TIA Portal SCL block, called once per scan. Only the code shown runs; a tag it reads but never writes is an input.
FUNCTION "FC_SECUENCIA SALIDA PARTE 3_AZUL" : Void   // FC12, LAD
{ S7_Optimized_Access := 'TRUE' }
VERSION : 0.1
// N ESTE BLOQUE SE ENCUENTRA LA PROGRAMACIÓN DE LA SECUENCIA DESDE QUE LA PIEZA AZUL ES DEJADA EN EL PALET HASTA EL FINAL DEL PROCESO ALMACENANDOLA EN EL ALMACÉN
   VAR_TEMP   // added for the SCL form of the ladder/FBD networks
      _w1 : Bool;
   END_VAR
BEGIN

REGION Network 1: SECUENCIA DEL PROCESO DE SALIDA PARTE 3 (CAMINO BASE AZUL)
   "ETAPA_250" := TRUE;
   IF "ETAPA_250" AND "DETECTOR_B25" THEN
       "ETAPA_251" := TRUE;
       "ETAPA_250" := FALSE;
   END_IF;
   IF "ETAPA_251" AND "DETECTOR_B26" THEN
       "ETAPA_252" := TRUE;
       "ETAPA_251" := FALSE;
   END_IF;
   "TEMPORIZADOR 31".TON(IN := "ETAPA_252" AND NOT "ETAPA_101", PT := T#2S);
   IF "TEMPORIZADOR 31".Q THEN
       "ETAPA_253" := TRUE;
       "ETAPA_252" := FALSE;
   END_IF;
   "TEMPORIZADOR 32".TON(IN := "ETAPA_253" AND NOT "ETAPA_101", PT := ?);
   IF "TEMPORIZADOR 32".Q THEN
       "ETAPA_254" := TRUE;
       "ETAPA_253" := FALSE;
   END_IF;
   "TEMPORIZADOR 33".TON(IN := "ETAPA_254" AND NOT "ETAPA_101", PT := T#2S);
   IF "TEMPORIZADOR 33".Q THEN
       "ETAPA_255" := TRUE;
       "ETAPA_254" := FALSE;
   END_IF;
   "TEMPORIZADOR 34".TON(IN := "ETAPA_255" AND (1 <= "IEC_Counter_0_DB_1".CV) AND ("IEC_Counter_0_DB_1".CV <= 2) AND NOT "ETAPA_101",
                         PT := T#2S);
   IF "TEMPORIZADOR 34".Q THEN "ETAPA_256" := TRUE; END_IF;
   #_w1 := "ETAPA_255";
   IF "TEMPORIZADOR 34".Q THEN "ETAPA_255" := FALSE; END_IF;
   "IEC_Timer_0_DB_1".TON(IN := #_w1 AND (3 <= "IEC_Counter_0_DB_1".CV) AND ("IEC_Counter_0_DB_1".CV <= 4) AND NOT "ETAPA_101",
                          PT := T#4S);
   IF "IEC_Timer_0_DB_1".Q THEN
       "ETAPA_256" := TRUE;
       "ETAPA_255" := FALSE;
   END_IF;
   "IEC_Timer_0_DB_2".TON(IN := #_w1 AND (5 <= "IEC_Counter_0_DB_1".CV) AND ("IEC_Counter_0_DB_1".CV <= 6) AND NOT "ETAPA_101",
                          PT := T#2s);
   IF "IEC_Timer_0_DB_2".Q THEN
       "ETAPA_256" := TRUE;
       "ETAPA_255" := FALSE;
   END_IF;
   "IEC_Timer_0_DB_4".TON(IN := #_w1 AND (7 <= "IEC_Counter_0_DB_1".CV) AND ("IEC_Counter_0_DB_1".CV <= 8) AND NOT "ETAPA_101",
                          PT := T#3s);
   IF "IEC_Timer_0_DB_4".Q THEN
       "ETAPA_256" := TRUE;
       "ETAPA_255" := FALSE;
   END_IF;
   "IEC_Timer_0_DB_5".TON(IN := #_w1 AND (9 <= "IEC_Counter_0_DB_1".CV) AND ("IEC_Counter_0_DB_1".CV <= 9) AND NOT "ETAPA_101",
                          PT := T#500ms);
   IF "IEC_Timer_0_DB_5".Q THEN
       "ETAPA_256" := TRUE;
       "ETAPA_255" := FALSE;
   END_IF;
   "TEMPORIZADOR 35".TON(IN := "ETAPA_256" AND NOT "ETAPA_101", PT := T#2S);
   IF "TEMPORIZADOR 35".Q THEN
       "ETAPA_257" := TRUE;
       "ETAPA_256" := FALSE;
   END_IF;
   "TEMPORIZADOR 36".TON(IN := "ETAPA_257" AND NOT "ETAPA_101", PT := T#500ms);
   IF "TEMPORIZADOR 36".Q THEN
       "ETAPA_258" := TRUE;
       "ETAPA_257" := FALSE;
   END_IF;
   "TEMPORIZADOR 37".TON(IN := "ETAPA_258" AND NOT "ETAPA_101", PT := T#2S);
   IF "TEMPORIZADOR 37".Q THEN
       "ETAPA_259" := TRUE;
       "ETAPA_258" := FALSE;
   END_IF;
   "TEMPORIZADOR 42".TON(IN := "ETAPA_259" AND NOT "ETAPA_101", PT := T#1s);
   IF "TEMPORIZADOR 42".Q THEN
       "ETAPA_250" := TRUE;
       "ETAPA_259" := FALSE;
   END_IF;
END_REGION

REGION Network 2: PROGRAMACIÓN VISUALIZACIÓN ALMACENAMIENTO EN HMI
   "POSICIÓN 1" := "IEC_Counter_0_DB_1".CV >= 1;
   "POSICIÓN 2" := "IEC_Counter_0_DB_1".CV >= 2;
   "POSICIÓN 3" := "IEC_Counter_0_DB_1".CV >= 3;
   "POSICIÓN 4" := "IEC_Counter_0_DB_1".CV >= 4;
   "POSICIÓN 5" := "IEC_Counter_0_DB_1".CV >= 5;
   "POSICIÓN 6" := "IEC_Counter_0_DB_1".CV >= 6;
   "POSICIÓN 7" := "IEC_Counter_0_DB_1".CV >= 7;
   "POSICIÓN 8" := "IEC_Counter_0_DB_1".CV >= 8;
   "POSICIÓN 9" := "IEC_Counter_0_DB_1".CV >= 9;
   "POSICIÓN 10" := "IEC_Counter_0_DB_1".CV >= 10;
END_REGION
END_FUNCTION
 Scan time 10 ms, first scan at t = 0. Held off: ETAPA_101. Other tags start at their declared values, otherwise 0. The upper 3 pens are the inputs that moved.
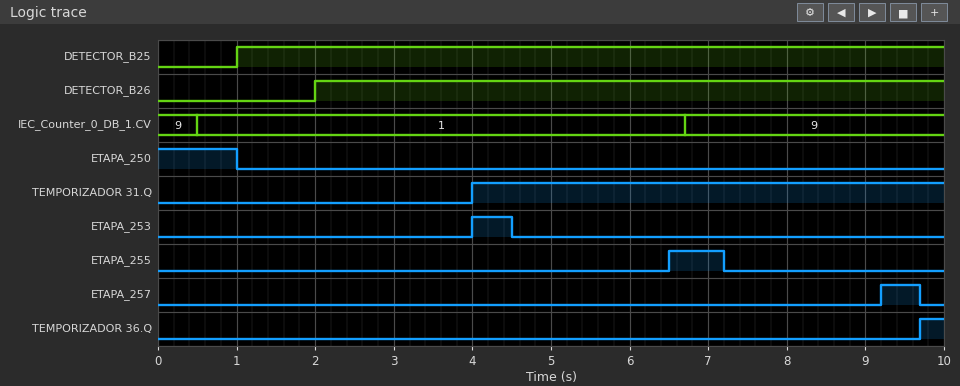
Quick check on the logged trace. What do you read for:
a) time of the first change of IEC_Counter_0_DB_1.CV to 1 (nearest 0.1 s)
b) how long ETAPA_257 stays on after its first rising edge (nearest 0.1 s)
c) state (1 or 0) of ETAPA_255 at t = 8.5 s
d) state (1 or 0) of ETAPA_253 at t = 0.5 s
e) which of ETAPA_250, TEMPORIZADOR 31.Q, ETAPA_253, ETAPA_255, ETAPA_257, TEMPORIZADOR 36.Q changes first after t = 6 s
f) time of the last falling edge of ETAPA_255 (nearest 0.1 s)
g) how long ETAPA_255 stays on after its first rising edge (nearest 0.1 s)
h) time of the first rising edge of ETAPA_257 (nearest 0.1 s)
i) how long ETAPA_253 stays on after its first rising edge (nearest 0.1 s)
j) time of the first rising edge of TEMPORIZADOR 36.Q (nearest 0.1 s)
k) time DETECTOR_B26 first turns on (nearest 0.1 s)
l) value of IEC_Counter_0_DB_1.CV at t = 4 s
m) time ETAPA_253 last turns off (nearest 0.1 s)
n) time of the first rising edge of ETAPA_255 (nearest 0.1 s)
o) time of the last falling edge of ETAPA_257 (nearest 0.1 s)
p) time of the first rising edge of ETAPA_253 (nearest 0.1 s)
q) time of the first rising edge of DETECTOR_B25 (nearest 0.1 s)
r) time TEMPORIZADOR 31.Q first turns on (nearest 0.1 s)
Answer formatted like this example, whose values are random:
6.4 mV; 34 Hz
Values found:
0.5 s; 0.5 s; 0; 0; ETAPA_255; 7.2 s; 0.7 s; 9.2 s; 0.5 s; 9.7 s; 2.0 s; 1; 4.5 s; 6.5 s; 9.7 s; 4.0 s; 1.0 s; 4.0 s
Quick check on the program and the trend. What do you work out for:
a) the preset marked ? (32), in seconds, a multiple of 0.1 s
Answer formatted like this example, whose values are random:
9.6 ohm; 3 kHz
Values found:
0.5 s
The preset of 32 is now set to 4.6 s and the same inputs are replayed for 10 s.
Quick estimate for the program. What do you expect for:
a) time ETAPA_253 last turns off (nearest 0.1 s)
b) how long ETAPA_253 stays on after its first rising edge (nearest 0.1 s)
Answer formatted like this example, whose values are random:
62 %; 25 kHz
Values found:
8.6 s; 4.6 s
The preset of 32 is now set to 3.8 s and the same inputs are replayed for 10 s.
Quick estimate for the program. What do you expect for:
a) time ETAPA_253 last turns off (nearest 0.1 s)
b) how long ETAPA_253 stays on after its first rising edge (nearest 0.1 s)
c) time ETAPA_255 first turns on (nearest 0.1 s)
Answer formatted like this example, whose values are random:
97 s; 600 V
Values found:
7.8 s; 3.8 s; 9.8 s
